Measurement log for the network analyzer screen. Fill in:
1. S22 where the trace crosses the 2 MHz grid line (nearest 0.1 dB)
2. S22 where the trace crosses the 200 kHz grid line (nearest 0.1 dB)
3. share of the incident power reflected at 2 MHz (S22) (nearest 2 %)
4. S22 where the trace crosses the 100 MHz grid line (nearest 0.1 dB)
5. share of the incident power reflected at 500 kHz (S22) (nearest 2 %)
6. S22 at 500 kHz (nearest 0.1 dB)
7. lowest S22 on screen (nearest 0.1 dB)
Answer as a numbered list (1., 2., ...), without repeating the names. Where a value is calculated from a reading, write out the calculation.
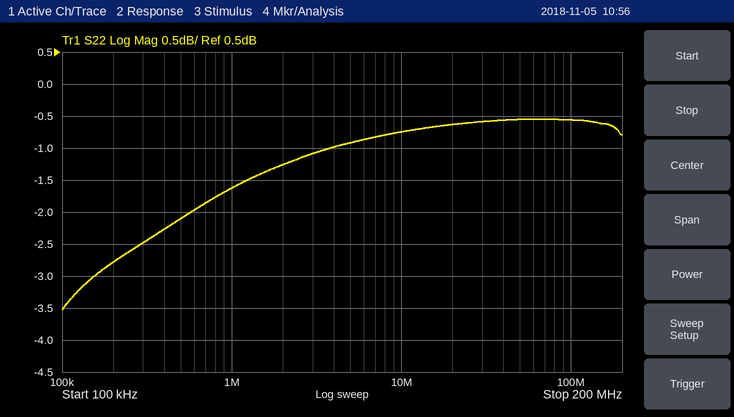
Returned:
1. -1.3 dB
2. -2.8 dB
3. 10^(-1.3/10) ≈ 74 %
4. -0.6 dB
5. 10^(-2.1/10) ≈ 62 %
6. -2.1 dB
7. -3.5 dB
